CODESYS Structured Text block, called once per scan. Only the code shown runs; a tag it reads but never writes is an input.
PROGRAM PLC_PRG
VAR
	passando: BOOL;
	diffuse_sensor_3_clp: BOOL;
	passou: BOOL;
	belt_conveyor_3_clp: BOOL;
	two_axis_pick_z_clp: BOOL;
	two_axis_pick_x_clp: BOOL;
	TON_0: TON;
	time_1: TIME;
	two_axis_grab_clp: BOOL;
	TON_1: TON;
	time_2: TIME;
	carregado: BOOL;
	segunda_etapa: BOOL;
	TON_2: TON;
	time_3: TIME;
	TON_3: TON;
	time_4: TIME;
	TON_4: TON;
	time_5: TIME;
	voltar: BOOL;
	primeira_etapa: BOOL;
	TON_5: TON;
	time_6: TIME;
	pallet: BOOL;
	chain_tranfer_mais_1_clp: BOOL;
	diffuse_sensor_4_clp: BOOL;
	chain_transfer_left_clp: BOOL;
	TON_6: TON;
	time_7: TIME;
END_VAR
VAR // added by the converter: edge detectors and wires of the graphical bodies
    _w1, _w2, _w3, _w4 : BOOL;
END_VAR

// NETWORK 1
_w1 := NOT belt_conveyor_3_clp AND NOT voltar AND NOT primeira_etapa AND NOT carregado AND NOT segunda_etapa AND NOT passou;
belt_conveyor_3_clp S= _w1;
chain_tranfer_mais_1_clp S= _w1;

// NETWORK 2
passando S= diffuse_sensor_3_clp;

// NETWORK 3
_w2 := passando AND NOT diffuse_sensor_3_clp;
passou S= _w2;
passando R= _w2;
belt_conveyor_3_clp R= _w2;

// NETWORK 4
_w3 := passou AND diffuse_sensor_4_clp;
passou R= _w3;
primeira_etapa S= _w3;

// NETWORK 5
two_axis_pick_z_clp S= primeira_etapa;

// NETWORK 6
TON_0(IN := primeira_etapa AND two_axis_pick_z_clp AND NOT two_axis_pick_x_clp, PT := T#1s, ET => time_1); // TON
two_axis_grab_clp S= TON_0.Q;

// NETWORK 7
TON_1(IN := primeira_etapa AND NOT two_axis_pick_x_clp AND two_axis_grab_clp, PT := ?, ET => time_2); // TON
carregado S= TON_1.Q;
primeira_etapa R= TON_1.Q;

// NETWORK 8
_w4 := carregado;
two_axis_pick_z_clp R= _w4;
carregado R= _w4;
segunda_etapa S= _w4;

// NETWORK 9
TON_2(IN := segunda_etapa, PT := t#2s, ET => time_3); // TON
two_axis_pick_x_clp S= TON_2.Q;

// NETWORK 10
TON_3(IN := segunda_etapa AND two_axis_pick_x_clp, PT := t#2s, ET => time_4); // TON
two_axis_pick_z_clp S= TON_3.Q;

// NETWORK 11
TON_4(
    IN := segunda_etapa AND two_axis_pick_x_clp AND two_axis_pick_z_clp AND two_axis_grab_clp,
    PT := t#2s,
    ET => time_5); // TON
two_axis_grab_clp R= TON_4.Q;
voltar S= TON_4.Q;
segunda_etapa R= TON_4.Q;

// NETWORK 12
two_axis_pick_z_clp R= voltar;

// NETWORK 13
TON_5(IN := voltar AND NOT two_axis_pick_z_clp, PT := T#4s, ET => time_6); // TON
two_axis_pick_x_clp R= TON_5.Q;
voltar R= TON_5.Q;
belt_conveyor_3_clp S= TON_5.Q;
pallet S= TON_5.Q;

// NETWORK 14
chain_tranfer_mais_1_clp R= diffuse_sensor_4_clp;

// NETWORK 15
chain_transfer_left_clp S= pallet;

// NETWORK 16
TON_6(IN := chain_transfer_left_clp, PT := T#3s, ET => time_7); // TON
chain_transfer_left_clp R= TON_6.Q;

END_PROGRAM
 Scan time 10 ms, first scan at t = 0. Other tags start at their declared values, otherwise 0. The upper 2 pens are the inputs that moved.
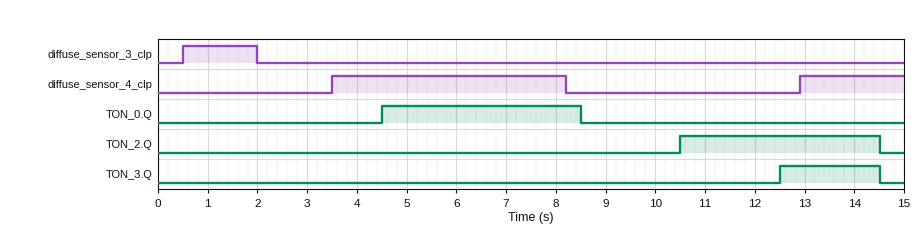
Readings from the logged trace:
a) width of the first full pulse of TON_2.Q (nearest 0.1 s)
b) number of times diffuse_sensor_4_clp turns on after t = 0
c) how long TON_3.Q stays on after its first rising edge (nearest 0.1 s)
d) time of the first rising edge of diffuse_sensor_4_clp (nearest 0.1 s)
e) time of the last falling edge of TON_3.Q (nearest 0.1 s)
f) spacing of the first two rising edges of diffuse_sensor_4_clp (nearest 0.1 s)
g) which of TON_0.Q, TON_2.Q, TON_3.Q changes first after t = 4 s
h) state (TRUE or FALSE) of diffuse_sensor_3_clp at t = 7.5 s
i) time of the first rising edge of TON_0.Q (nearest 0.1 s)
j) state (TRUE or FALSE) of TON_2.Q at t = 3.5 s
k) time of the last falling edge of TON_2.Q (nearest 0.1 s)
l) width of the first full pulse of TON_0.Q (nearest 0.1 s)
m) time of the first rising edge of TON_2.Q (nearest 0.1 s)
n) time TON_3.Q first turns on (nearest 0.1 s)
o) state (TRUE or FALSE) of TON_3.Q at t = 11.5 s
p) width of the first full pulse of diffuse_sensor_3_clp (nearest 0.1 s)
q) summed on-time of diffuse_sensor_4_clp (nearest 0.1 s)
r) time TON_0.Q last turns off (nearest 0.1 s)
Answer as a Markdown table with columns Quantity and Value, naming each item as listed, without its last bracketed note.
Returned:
| Quantity | Value |
|---|---|
| width of the first full pulse of TON_2.Q | 4.0 s |
| number of times diffuse_sensor_4_clp turns on after t = 0 | 2 |
| how long TON_3.Q stays on after its first rising edge | 2.0 s |
| time of the first rising edge of diffuse_sensor_4_clp | 3.5 s |
| time of the last falling edge of TON_3.Q | 14.5 s |
| spacing of the first two rising edges of diffuse_sensor_4_clp | 9.4 s |
| which of TON_0.Q, TON_2.Q, TON_3.Q changes first after t = 4 s | TON_0.Q |
| state (TRUE or FALSE) of diffuse_sensor_3_clp at t = 7.5 s | FALSE |
| time of the first rising edge of TON_0.Q | 4.5 s |
| state (TRUE or FALSE) of TON_2.Q at t = 3.5 s | FALSE |
| time of the last falling edge of TON_2.Q | 14.5 s |
| width of the first full pulse of TON_0.Q | 4.0 s |
| time of the first rising edge of TON_2.Q | 10.5 s |
| time TON_3.Q first turns on | 12.5 s |
| state (TRUE or FALSE) of TON_3.Q at t = 11.5 s | FALSE |
| width of the first full pulse of diffuse_sensor_3_clp | 1.5 s |
| summed on-time of diffuse_sensor_4_clp | 6.8 s |
| time TON_0.Q last turns off | 8.5 s |
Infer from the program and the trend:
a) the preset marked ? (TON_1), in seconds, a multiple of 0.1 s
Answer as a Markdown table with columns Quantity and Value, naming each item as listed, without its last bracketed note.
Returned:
| Quantity | Value |
|---|---|
| the preset marked ? (TON_1), in seconds, a multiple of 0.1 s | 4.0 s |
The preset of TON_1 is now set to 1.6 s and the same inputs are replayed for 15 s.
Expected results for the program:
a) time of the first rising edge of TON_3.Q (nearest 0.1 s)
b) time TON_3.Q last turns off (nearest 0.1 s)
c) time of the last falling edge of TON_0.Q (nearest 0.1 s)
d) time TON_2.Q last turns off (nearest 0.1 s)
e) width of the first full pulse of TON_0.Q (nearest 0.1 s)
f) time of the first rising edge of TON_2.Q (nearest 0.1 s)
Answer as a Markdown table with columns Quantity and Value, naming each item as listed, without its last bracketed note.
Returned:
| Quantity | Value |
|---|---|
| time of the first rising edge of TON_3.Q | 10.1 s |
| time TON_3.Q last turns off | 12.1 s |
| time of the last falling edge of TON_0.Q | 6.1 s |
| time TON_2.Q last turns off | 12.1 s |
| width of the first full pulse of TON_0.Q | 1.6 s |
| time of the first rising edge of TON_2.Q | 8.1 s |
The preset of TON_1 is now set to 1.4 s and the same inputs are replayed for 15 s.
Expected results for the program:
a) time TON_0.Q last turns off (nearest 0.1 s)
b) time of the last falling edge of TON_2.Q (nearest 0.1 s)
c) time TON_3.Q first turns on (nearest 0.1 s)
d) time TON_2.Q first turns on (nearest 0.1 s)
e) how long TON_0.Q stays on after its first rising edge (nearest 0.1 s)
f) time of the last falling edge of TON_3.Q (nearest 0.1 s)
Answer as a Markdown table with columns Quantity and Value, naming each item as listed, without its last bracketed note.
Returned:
| Quantity | Value |
|---|---|
| time TON_0.Q last turns off | 5.9 s |
| time of the last falling edge of TON_2.Q | 11.9 s |
| time TON_3.Q first turns on | 9.9 s |
| time TON_2.Q first turns on | 7.9 s |
| how long TON_0.Q stays on after its first rising edge | 1.4 s |
| time of the last falling edge of TON_3.Q | 11.9 s |
